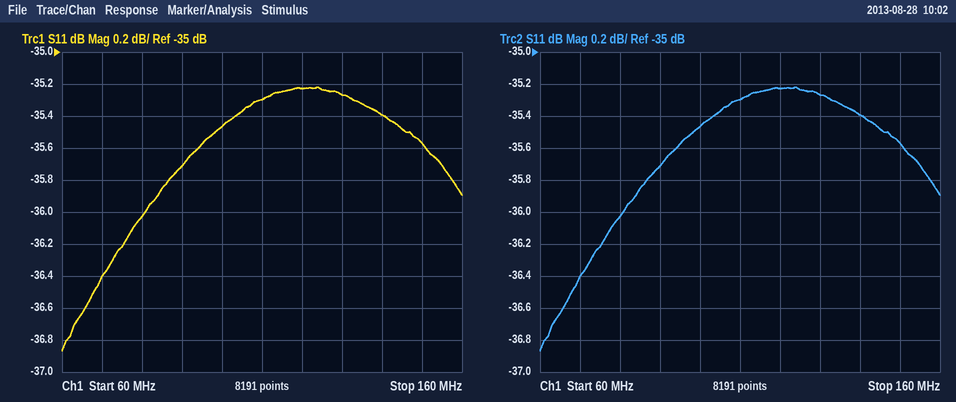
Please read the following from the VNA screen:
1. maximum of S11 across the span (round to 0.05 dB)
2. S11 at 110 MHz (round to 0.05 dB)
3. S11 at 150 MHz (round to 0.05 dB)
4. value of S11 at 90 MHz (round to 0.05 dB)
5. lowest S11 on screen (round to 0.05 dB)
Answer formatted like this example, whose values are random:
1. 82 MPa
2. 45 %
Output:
1. -35.20 dB
2. -35.30 dB
3. -35.55 dB
4. -35.70 dB
5. -36.85 dB
